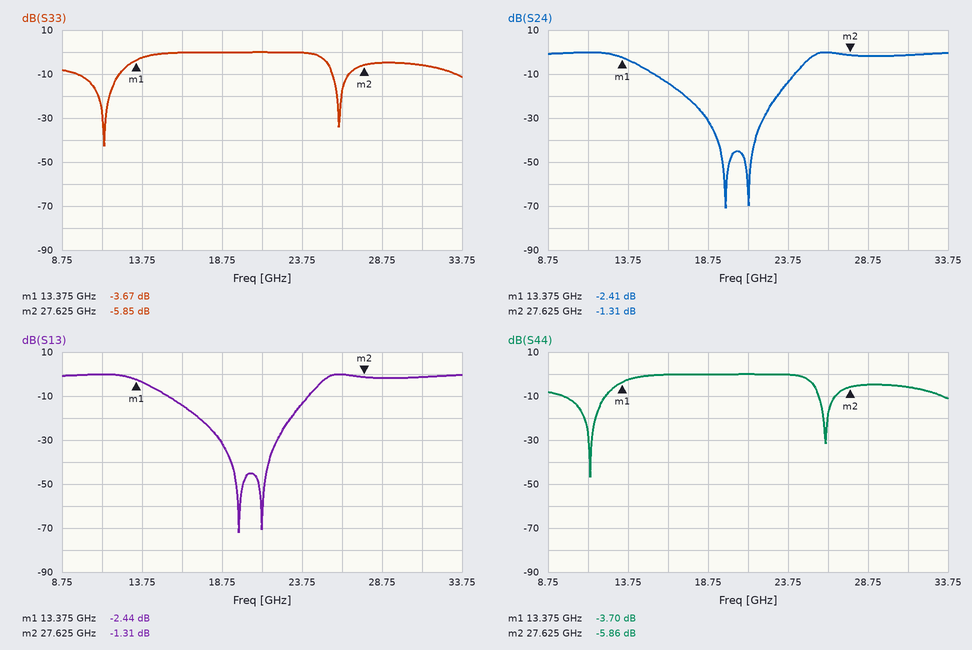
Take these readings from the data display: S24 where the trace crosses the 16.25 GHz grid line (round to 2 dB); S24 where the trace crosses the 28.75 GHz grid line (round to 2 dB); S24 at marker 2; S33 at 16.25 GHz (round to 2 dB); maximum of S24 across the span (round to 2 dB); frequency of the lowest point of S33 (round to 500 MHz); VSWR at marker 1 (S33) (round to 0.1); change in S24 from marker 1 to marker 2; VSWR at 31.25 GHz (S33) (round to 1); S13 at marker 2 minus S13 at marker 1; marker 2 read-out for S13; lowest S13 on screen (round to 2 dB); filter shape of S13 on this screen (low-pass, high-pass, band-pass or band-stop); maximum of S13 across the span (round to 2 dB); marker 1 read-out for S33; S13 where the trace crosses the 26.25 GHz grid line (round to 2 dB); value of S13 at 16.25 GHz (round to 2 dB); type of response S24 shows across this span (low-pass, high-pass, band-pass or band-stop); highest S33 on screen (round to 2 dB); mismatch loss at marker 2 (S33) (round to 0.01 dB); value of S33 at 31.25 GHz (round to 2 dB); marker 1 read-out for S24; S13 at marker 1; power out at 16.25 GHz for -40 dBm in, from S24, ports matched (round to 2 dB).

-14 dB
-2 dB
-1.31 dB
0 dB
0 dB
11.5 GHz
4.8
1.10 dB
3
1.13 dB
-1.31 dB
-72 dB
band-stop
0 dB
-3.67 dB
0 dB
-14 dB
band-stop
0 dB
1.31 dB
-6 dB
-2.41 dB
-2.44 dB
-54 dBm
